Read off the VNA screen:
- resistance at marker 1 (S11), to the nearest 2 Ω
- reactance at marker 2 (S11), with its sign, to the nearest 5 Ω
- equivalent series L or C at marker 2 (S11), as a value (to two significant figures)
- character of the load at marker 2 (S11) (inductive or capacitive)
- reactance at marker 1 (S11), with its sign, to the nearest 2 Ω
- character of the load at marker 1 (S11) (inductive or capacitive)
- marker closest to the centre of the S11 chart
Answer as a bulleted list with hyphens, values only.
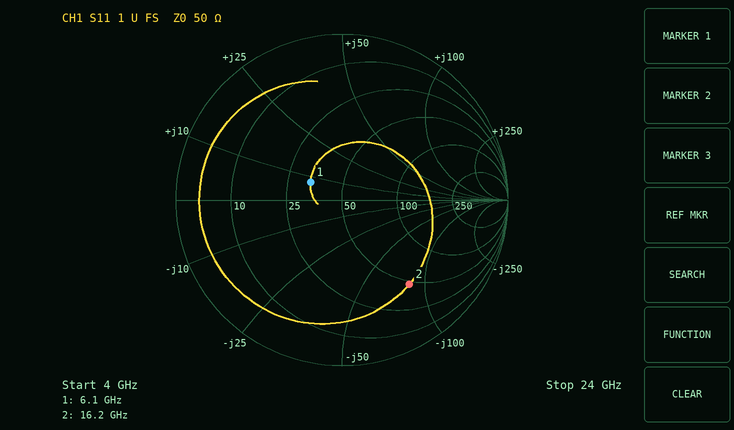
- 34 Ω
- -85 Ω
- 120 fF
- capacitive
- +8 Ω
- inductive
- marker 1
